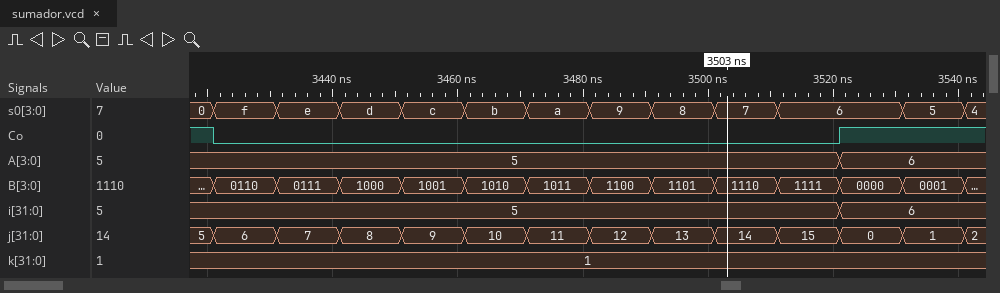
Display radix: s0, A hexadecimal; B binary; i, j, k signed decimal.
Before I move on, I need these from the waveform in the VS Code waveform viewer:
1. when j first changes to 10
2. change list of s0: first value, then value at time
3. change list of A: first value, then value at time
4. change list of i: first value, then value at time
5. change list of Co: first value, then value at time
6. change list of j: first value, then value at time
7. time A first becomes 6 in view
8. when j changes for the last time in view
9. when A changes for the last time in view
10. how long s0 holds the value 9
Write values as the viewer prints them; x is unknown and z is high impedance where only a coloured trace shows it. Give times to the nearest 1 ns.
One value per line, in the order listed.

3461 ns
0, f at 3421 ns, e at 3431 ns, d at 3441 ns, c at 3451 ns, b at 3461 ns, a at 3471 ns, 9 at 3481 ns, 8 at 3491 ns, 7 at 3501 ns, 6 at 3511 ns, 5 at 3531 ns, 4 at 3541 ns
5, 6 at 3521 ns
5, 6 at 3521 ns
1, 0 at 3421 ns, 1 at 3521 ns
5, 6 at 3421 ns, 7 at 3431 ns, 8 at 3441 ns, 9 at 3451 ns, 10 at 3461 ns, 11 at 3471 ns, 12 at 3481 ns, 13 at 3491 ns, 14 at 3501 ns, 15 at 3511 ns, 0 at 3521 ns, 1 at 3531 ns, 2 at 3541 ns
3521 ns
3541 ns
3521 ns
10 ns
